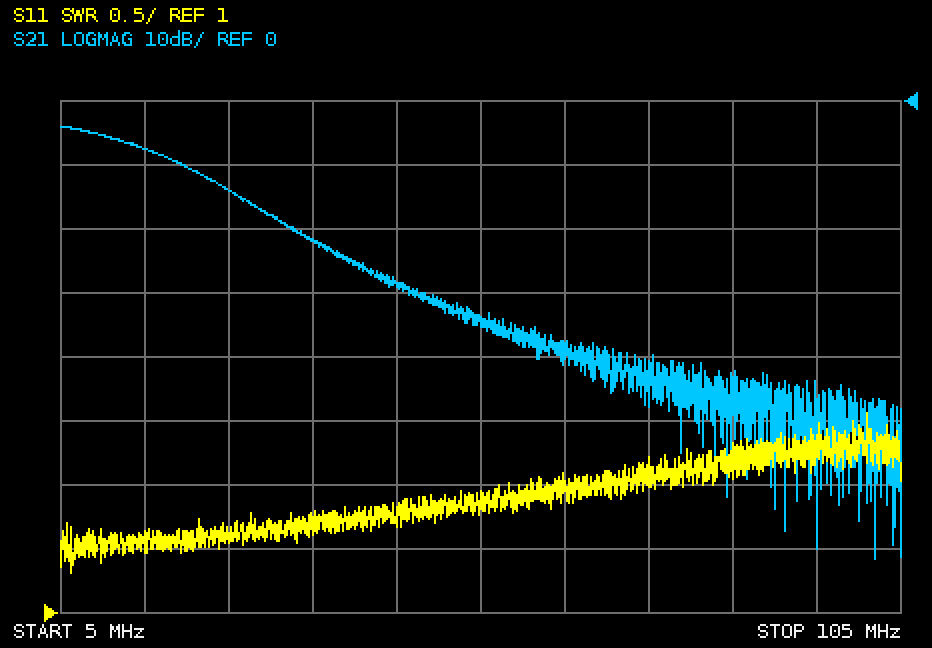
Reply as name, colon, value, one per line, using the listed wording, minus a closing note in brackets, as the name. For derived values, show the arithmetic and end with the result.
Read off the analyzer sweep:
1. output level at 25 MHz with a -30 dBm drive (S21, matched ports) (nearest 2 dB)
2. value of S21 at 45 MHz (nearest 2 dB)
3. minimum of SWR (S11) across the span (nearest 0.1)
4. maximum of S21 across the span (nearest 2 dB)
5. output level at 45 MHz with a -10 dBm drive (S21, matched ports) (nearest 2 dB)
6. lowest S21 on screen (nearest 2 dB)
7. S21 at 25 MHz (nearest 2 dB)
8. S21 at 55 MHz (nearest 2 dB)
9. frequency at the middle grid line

output level at 25 MHz with a -30 dBm drive (S21, matched ports): -30 dBm + (-14 dB) = -44 dBm
value of S21 at 45 MHz: -28 dB
minimum of SWR (S11) across the span: 1.3
maximum of S21 across the span: -4 dB
output level at 45 MHz with a -10 dBm drive (S21, matched ports): -10 dBm + (-28 dB) = -38 dBm
lowest S21 on screen: -72 dB
S21 at 25 MHz: -14 dB
S21 at 55 MHz: -34 dB
frequency at the middle grid line: 55 MHz
